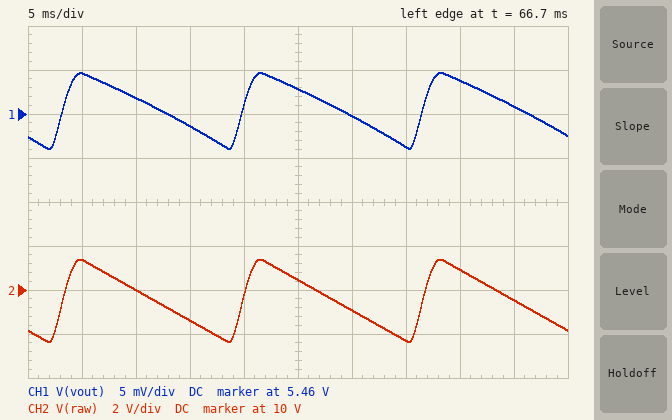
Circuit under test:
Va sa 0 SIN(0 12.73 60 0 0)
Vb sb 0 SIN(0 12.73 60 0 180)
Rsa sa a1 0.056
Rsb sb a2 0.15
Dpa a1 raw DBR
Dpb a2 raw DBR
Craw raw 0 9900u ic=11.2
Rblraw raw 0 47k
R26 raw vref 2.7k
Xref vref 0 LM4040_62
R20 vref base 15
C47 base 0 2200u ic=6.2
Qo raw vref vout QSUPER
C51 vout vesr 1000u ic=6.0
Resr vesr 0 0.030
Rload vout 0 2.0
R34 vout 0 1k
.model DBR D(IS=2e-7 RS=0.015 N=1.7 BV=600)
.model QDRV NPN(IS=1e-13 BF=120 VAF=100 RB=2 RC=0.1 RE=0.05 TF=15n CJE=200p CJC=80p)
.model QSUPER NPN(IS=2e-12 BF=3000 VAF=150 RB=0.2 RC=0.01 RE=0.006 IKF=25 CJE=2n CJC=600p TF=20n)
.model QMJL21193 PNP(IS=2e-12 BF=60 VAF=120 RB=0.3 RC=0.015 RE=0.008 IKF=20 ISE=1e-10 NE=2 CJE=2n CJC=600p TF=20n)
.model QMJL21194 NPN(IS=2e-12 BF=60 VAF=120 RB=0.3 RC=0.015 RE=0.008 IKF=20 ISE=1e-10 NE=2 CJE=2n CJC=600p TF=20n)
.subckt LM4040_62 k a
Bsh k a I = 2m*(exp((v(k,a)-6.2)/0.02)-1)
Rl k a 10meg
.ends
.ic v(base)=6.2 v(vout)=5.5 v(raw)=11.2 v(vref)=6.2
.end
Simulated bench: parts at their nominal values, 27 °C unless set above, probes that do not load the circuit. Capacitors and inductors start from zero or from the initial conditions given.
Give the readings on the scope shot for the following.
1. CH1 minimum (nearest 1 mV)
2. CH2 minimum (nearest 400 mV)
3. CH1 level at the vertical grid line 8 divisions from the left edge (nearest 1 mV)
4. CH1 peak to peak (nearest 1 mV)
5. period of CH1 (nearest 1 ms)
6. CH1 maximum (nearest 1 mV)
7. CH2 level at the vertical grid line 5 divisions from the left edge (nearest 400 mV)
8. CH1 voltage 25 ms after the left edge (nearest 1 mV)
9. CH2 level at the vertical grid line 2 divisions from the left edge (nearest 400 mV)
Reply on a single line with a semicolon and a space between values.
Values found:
5.456 V; 7.6 V; 5.464 V; 9 mV; 17 ms; 5.465 V; 10.4 V; 5.463 V; 10.0 V
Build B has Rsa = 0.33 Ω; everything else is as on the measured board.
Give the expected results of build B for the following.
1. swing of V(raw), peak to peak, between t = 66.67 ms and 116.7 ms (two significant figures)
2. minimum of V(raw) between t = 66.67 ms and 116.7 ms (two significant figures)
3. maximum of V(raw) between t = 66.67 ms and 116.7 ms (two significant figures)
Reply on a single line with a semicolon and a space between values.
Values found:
3.2 V; 5.2 V; 8.5 V
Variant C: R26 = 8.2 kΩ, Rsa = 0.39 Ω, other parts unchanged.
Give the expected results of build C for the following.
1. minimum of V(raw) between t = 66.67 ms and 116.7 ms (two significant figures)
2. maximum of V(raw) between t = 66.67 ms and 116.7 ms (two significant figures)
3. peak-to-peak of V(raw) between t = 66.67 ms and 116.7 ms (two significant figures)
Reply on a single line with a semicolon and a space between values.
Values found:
4.9 V; 8.0 V; 3.1 V
